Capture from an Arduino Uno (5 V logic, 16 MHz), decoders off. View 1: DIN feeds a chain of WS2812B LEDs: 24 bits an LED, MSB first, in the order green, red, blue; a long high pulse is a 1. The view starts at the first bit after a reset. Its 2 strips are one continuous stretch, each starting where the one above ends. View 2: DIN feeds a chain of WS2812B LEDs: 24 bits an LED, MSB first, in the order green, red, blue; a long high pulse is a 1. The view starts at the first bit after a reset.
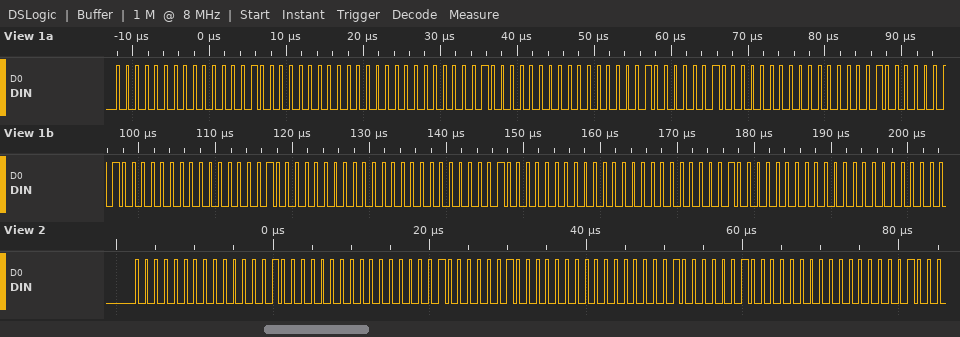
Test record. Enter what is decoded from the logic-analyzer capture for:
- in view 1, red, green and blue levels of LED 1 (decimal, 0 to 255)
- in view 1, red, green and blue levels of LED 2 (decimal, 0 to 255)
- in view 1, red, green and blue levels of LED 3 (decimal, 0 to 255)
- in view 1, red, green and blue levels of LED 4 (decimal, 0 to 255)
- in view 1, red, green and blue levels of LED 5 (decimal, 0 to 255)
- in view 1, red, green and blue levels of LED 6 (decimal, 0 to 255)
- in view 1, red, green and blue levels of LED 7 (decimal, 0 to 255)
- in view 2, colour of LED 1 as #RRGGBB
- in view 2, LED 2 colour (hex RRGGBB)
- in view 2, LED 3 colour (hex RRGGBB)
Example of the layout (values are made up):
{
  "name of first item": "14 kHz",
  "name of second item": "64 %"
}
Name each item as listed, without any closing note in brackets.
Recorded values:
{
  "in view 1, red, green and blue levels of LED 1": "2, 0, 0",
  "in view 1, red, green and blue levels of LED 2": "2, 0, 0",
  "in view 1, red, green and blue levels of LED 3": "2, 1, 0",
  "in view 1, red, green and blue levels of LED 4": "1, 1, 0",
  "in view 1, red, green and blue levels of LED 5": "0, 1, 0",
  "in view 1, red, green and blue levels of LED 6": "0, 1, 0",
  "in view 1, red, green and blue levels of LED 7": "0, 1, 0",
  "in view 2, colour of LED 1 as #RRGGBB": "#020000",
  "in view 2, LED 2 colour": "#020100",
  "in view 2, LED 3 colour": "#020100"
}
